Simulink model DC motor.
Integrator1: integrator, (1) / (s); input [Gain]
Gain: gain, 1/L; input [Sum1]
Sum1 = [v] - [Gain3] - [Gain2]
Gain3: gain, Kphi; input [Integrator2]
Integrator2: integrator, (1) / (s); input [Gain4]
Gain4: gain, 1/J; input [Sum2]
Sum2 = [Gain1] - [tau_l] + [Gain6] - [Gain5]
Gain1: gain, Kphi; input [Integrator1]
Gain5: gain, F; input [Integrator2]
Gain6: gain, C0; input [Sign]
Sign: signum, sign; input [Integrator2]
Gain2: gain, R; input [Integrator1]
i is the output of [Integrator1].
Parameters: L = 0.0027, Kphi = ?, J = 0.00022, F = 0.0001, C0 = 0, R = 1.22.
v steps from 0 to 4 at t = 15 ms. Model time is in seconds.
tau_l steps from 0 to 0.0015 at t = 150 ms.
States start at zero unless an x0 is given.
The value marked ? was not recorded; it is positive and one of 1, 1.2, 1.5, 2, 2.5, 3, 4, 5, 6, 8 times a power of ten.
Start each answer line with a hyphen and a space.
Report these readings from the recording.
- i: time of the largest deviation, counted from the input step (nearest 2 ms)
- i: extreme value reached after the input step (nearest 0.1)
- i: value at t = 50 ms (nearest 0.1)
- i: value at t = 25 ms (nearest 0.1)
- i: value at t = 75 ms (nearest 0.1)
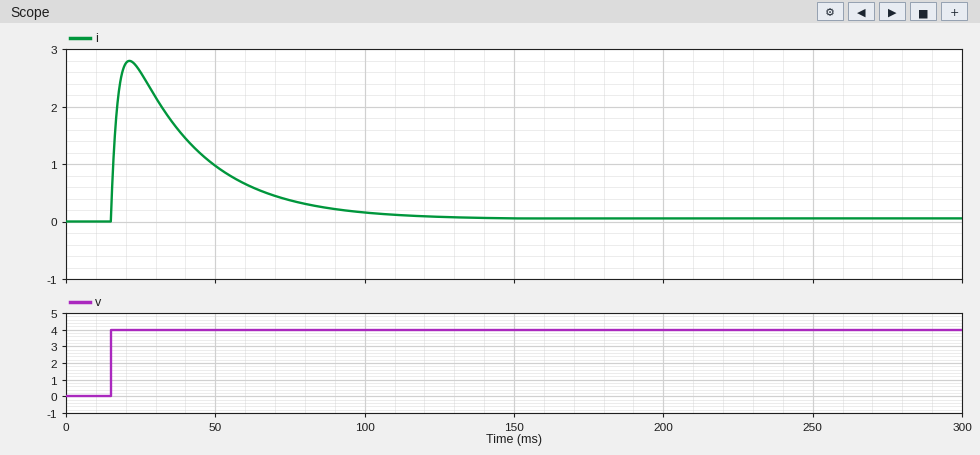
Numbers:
- 6 ms
- 2.8
- 1.0
- 2.6
- 0.4
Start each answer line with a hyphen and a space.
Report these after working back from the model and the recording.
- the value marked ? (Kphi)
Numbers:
- 0.1
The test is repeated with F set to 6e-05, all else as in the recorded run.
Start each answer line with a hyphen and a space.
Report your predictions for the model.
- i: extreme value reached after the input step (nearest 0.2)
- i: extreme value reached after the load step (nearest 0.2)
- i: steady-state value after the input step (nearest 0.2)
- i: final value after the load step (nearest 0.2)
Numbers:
- 2.8
- 0.0
- 0.0
- 0.0
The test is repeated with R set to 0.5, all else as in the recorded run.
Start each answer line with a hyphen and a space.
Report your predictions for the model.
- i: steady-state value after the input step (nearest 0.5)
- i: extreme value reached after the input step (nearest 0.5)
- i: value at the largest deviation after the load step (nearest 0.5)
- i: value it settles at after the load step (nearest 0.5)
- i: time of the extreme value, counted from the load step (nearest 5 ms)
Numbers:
- 0.0
- 5.0
- 0.0
- 0.0
- 35 ms
